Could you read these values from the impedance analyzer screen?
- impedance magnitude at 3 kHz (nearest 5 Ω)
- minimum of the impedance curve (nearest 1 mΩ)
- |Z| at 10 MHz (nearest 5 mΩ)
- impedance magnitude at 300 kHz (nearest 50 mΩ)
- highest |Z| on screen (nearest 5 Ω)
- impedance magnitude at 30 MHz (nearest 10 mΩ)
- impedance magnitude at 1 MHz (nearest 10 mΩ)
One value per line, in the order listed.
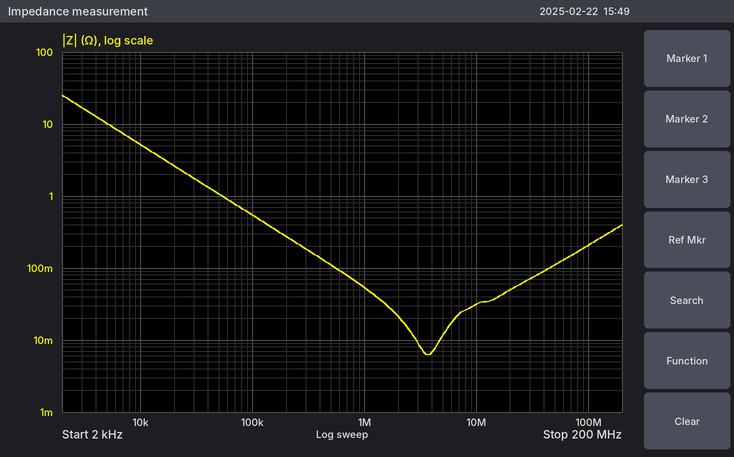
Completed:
15 Ω
6 mΩ
30 mΩ
200 mΩ
25 Ω
70 mΩ
50 mΩ
